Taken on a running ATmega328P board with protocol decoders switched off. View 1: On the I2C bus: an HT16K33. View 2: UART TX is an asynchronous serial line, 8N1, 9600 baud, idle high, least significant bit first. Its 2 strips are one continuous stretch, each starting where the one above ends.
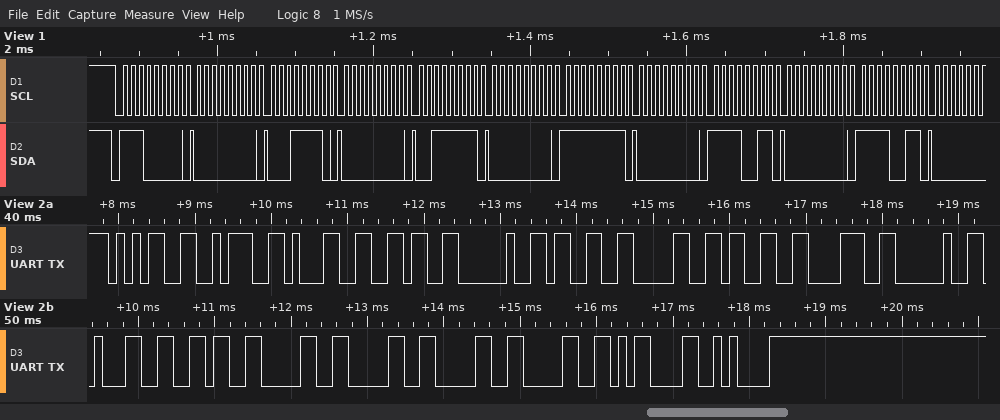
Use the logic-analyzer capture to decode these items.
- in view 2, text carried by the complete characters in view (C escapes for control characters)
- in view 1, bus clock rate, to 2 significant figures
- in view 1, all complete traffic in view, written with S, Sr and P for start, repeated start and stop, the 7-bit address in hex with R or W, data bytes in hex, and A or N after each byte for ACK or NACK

"5:16 3038 160000\r\n"
100 kHz
S 70W A 00 A 1E A 00 A 3F A 00 A FF A 00 A F3 A 00 A F3 A
